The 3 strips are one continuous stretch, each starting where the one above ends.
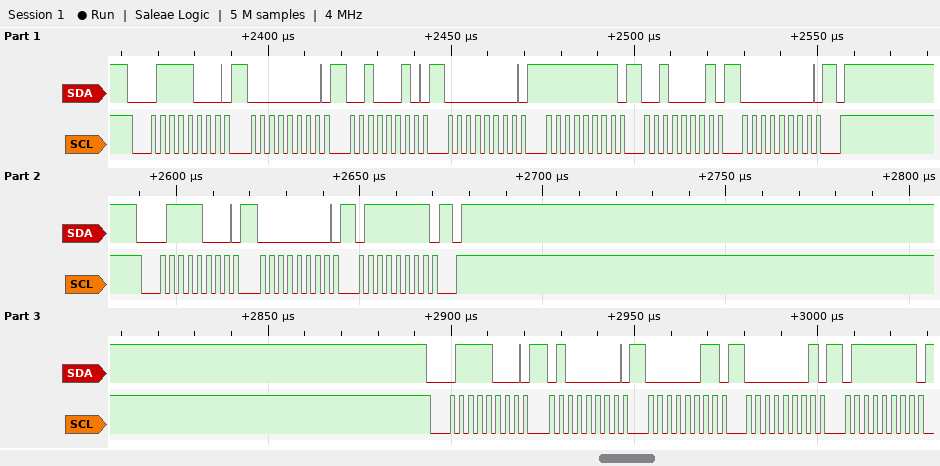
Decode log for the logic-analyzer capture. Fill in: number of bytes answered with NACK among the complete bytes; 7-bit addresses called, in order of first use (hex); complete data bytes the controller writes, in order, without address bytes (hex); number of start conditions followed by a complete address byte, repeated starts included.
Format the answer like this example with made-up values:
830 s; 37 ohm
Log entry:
0; 0x3C; 00 22 00 FF 21 00 00 7F 40 03 01 7F; 3
